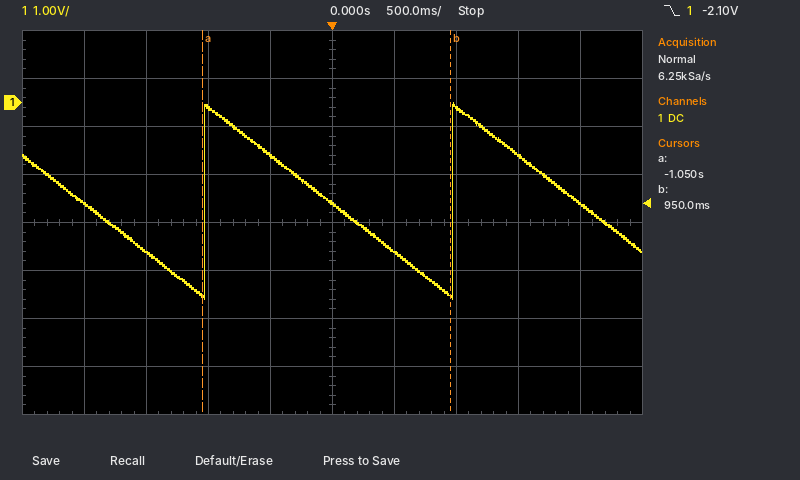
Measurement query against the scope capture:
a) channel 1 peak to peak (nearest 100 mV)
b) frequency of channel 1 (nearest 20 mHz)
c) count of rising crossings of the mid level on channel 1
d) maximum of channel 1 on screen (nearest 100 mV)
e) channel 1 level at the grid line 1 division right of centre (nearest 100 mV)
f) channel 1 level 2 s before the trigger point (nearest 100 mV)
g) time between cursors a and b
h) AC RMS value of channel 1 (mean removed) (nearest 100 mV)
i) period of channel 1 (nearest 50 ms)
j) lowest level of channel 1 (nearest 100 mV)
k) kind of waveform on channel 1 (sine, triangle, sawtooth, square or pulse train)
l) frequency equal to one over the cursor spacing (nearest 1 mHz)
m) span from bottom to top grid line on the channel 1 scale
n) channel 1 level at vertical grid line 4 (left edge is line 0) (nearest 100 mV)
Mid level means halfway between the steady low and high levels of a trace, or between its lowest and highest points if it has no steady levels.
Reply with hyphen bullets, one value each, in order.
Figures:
- 4.1 V
- 500 mHz
- 2
- 0.0 V
- -3.1 V
- -2.1 V
- 2.00 s
- 1.2 V
- 2.00 s
- -4.1 V
- sawtooth
- 500 mHz
- 8 V
- -1.1 V
